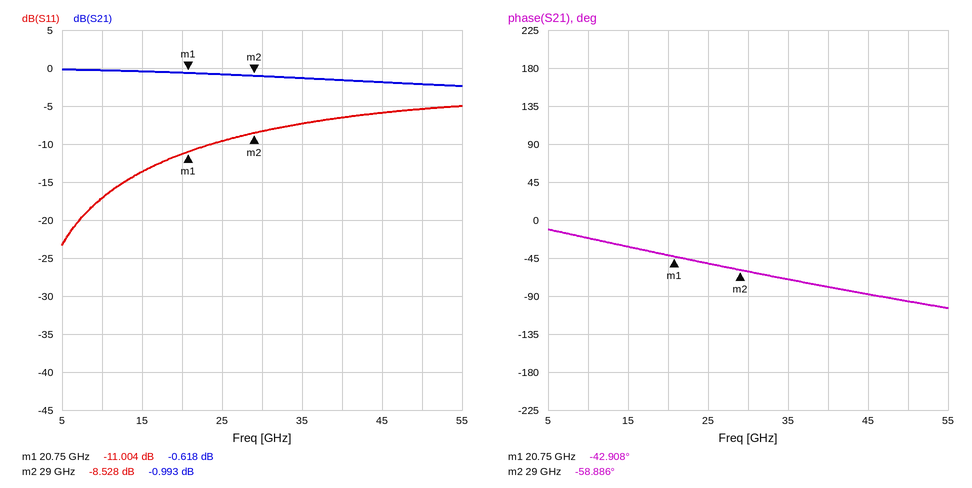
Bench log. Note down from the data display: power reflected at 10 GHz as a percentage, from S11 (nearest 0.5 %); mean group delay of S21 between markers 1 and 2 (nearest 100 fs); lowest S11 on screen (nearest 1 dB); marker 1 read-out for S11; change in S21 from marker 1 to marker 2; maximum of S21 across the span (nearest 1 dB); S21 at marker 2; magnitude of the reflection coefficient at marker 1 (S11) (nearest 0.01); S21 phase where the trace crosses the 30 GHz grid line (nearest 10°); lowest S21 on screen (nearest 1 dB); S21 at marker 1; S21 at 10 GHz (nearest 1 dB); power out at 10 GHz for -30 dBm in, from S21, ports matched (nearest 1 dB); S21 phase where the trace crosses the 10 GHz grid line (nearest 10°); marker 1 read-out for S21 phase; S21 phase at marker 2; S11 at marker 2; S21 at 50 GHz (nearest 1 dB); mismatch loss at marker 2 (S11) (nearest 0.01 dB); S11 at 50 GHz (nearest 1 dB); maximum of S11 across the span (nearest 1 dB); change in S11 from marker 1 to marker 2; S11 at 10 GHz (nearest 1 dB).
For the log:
2.0 %
5.4 ps
-23 dB
-11.004 dB
-0.375 dB
0 dB
-0.993 dB
0.28
-60°
-2 dB
-0.618 dB
0 dB
-30 dBm
-20°
-42.908°
-58.886°
-8.528 dB
-2 dB
0.66 dB
-5 dB
-5 dB
2.476 dB
-17 dB
